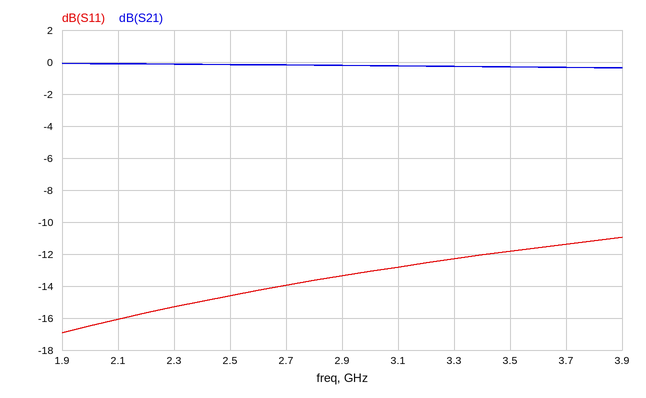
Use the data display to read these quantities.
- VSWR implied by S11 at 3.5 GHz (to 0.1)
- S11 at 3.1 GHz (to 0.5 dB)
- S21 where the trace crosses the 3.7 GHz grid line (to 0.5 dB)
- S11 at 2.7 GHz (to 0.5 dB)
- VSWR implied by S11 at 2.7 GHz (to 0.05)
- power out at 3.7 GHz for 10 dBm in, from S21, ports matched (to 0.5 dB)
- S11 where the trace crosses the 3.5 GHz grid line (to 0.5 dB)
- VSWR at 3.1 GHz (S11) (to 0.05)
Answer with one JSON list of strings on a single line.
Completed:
["1.7", "-13.0 dB", "-0.5 dB", "-14.0 dB", "1.50", "9.5 dBm", "-12.0 dB", "1.60"]
